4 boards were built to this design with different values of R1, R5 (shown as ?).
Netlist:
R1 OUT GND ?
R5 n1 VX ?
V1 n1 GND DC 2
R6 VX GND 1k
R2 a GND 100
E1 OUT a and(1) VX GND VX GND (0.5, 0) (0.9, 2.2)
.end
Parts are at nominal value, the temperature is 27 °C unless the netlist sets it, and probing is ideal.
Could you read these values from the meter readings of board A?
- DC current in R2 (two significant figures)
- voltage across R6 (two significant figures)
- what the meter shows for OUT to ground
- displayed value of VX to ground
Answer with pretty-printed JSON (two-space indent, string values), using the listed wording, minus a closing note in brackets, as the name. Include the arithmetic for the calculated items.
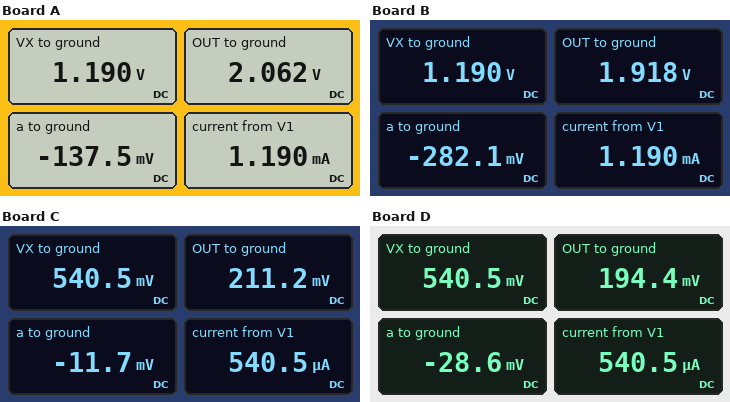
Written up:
{
  "DC current in R2": "(0 V - (-137.5 mV)) / 100 Ω = 1.4 mA",
  "voltage across R6": "1.19 V = 1.2 V",
  "what the meter shows for OUT to ground": "2.062 V",
  "displayed value of VX to ground": "1.190 V"
}
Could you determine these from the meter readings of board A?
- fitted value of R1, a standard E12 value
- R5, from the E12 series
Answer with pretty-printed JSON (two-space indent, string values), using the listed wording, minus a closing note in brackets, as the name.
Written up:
{
  "fitted value of R1, a standard E12 value": "1.5 kΩ",
  "R5, from the E12 series": "680 Ω"
}
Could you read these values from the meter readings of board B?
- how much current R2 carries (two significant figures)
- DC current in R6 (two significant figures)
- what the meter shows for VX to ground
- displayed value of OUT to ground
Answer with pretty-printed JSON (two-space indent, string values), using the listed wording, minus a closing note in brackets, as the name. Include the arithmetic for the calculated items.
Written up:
{
  "how much current R2 carries": "(0 V - (-282.1 mV)) / 100 Ω = 2.8 mA",
  "DC current in R6": "(1.19 V) / 1 kΩ = 1.2 mA",
  "what the meter shows for VX to ground": "1.190 V",
  "displayed value of OUT to ground": "1.918 V"
}
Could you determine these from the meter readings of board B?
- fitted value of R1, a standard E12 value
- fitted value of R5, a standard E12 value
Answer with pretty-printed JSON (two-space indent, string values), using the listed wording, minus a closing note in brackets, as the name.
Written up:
{
  "fitted value of R1, a standard E12 value": "680 Ω",
  "fitted value of R5, a standard E12 value": "680 Ω"
}
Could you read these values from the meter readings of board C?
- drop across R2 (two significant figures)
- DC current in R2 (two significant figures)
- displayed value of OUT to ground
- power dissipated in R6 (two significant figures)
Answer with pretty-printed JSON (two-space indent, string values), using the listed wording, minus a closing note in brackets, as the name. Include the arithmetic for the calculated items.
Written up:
{
  "drop across R2": "0 V - (-11.7 mV) = 12 mV",
  "DC current in R2": "(0 V - (-11.7 mV)) / 100 Ω = 120 µA",
  "displayed value of OUT to ground": "211.2 mV",
  "power dissipated in R6": "(540.5 mV)^2 / 1 kΩ = 290 µW"
}
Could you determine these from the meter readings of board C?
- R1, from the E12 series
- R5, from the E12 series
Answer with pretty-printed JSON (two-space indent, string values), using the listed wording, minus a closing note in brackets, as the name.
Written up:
{
  "R1, from the E12 series": "1.8 kΩ",
  "R5, from the E12 series": "2.7 kΩ"
}
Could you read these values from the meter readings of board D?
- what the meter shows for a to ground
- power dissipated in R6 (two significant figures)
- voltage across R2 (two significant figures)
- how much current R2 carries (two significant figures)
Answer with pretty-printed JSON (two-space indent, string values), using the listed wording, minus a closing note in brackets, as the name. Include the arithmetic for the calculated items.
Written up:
{
  "what the meter shows for a to ground": "-28.6 mV",
  "power dissipated in R6": "(540.5 mV)^2 / 1 kΩ = 290 µW",
  "voltage across R2": "0 V - (-28.6 mV) = 29 mV",
  "how much current R2 carries": "(0 V - (-28.6 mV)) / 100 Ω = 290 µA"
}
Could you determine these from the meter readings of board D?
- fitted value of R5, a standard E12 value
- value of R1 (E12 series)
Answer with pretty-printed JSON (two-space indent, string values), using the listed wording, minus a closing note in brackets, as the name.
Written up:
{
  "fitted value of R5, a standard E12 value": "2.7 kΩ",
  "value of R1": "680 Ω"
}
